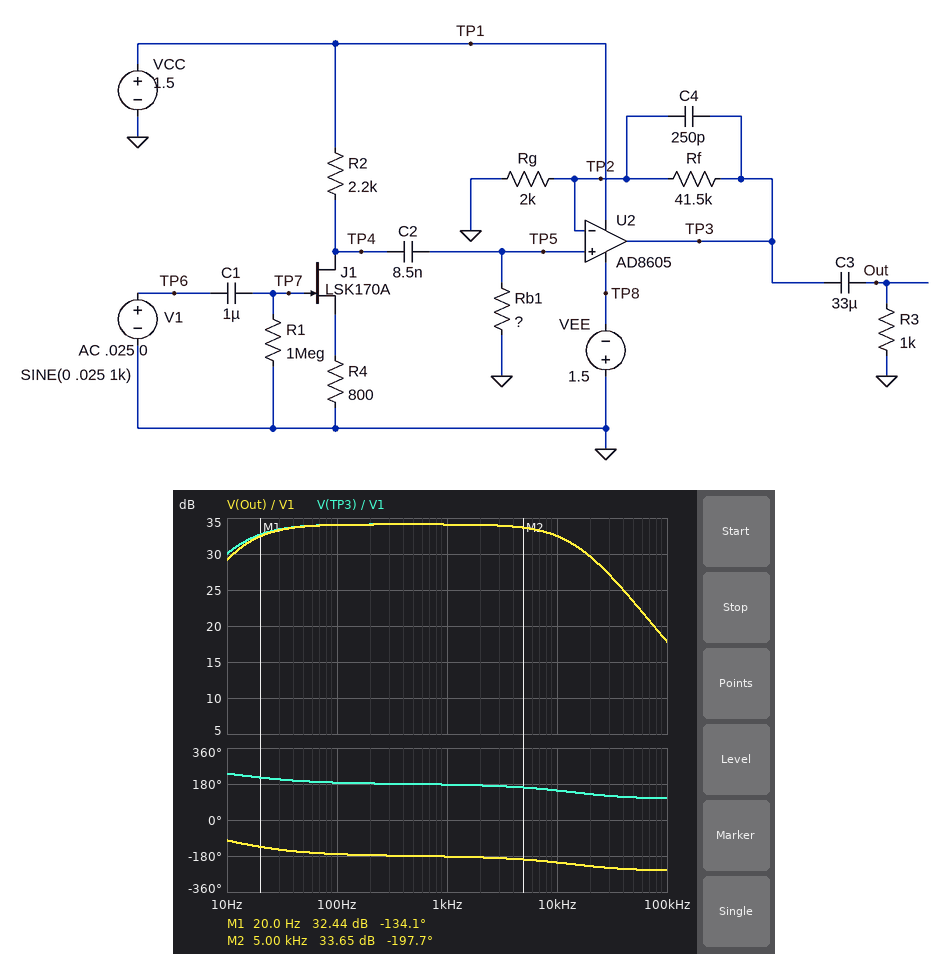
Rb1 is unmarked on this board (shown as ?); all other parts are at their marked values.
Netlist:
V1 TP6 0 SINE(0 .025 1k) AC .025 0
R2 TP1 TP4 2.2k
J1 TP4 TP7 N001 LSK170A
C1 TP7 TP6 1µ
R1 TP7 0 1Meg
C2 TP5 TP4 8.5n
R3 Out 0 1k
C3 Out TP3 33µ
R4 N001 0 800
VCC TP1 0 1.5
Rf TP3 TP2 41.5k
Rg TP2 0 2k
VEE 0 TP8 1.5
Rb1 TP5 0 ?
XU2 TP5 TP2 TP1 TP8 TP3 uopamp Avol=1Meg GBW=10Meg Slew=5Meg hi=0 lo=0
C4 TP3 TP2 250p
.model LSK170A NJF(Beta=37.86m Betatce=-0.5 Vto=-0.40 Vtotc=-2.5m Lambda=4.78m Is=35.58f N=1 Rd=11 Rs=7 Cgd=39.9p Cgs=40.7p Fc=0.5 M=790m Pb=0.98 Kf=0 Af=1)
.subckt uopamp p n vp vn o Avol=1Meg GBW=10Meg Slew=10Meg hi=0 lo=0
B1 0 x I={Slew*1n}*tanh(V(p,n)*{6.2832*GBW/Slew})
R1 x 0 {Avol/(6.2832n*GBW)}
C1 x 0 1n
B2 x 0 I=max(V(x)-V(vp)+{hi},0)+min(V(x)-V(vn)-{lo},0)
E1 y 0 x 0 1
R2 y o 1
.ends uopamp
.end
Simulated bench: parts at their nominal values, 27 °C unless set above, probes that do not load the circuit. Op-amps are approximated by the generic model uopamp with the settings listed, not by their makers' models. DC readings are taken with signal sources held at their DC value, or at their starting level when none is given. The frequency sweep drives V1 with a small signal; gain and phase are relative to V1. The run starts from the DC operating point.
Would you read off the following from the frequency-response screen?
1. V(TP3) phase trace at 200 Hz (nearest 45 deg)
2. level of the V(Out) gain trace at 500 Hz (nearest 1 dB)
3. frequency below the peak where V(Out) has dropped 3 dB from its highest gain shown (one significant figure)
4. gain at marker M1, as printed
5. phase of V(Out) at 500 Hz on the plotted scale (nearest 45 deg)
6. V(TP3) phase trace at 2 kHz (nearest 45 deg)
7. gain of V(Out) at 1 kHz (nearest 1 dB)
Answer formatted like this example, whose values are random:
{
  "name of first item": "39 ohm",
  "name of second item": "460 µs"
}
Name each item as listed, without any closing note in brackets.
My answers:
{
  "V(TP3) phase trace at 200 Hz": "180 deg",
  "level of the V(Out) gain trace at 500 Hz": "34 dB",
  "frequency below the peak where V(Out) has dropped 3 dB from its highest gain shown": "10 Hz",
  "gain at marker M1, as printed": "32.44 dB",
  "phase of V(Out) at 500 Hz on the plotted scale": "-180 deg",
  "V(TP3) phase trace at 2 kHz": "180 deg",
  "gain of V(Out) at 1 kHz": "34 dB"
}
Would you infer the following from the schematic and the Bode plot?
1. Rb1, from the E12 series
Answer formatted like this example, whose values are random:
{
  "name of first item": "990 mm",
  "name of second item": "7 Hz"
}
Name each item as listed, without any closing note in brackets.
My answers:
{
  "Rb1, from the E12 series": "1.5 MΩ"
}
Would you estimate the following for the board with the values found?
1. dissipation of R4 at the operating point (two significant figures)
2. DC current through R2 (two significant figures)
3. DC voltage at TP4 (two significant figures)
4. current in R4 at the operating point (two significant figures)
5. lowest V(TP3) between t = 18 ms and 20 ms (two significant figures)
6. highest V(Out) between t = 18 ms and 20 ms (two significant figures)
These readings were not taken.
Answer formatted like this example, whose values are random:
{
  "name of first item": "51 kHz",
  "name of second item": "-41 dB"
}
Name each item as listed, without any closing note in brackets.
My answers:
{
  "dissipation of R4 at the operating point": "110 µW",
  "DC current through R2": "370 µA",
  "DC voltage at TP4": "680 mV",
  "current in R4 at the operating point": "370 µA",
  "lowest V(TP3) between t = 18 ms and 20 ms": "-1.3 V",
  "highest V(Out) between t = 18 ms and 20 ms": "1.3 V"
}
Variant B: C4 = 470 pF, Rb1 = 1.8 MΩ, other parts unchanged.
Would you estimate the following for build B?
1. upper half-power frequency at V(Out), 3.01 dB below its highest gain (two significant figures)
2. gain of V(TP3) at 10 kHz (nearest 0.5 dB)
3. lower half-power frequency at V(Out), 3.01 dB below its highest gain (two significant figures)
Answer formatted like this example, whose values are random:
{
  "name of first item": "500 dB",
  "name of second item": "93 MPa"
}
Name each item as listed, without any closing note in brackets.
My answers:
{
  "upper half-power frequency at V(Out), 3.01 dB below its highest gain": "8.1 kHz",
  "gain of V(TP3) at 10 kHz": "30.0 dB",
  "lower half-power frequency at V(Out), 3.01 dB below its highest gain": "12 Hz"
}
